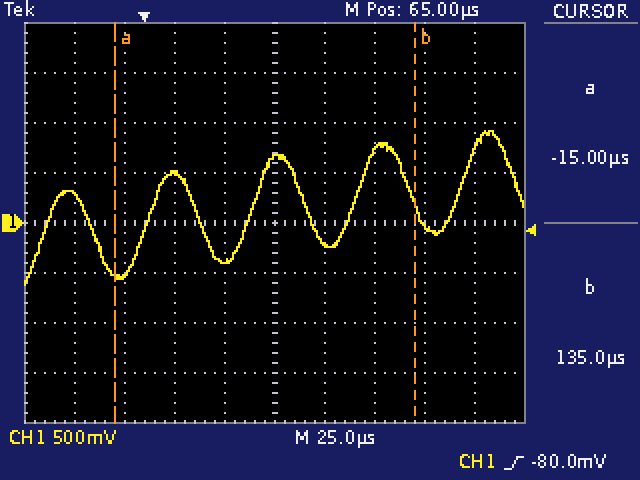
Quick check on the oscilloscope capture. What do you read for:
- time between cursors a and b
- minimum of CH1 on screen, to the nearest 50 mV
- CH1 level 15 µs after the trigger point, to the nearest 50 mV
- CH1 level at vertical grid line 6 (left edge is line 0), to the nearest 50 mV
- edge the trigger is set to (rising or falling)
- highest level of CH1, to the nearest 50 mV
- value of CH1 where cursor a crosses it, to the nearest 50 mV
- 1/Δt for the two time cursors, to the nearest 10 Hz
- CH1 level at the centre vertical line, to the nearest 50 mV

150.0 µs
-600 mV
500 mV
-200 mV
rising
900 mV
-500 mV
6.67 kHz
650 mV
